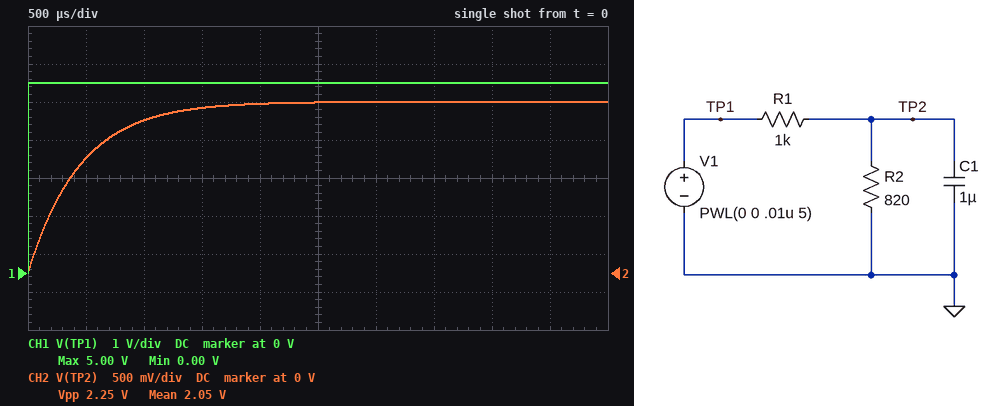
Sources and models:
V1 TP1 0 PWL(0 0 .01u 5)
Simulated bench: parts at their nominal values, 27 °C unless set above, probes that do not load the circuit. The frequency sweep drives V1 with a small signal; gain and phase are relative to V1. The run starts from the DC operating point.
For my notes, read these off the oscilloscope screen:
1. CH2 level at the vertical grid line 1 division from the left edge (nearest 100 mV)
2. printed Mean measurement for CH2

1.5 V
2.05 V
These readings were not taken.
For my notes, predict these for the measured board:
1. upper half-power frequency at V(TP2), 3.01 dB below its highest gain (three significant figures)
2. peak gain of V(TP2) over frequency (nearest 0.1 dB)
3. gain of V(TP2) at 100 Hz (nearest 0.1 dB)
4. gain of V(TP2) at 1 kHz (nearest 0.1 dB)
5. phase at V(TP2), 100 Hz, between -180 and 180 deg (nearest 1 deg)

353 Hz
-6.9 dB
-7.3 dB
-16.5 dB
-16 deg
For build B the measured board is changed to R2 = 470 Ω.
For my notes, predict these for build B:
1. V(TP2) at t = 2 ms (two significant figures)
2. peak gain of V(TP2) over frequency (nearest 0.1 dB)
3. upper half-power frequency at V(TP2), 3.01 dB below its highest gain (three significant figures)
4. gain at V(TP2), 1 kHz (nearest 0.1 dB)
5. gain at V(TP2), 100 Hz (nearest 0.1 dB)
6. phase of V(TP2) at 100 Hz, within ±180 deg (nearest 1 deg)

1.6 V
-9.9 dB
498 Hz
-16.9 dB
-10.1 dB
-11 deg
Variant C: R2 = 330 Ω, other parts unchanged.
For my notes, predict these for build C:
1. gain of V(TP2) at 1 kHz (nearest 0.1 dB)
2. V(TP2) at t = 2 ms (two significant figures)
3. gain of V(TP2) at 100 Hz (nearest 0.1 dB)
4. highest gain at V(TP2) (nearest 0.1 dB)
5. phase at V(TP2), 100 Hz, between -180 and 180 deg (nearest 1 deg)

-17.5 dB
1.2 V
-12.2 dB
-12.1 dB
-9 deg
